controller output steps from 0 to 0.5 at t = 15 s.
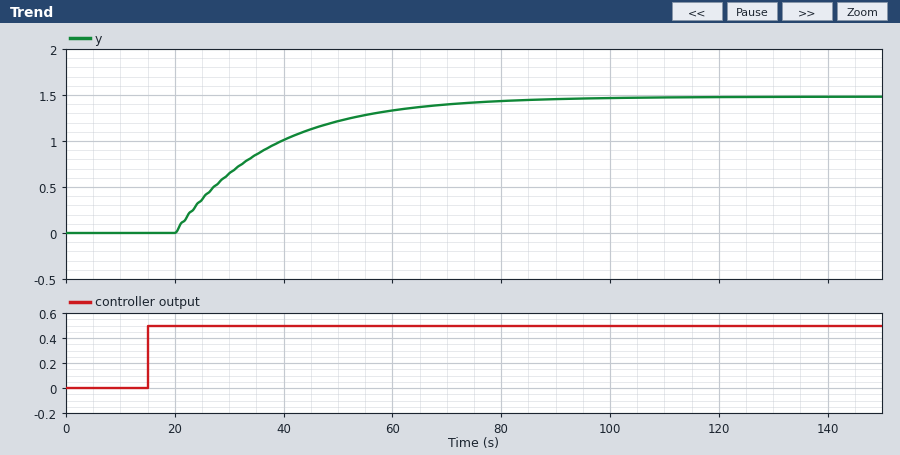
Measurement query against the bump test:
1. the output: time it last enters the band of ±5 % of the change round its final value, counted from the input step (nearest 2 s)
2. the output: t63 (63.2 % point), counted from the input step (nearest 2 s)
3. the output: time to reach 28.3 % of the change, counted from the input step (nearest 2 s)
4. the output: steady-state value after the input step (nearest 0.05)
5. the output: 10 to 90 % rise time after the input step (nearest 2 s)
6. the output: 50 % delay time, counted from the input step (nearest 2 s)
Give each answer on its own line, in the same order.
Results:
58 s
22 s
10 s
1.50
38 s
18 s
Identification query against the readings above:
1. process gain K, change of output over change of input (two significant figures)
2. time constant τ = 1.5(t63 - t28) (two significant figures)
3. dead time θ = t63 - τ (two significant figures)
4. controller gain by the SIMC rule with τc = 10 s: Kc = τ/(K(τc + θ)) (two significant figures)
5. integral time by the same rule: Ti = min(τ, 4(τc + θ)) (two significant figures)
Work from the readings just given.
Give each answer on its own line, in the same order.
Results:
3.0
18 s
4.0 s
0.43
18 s
